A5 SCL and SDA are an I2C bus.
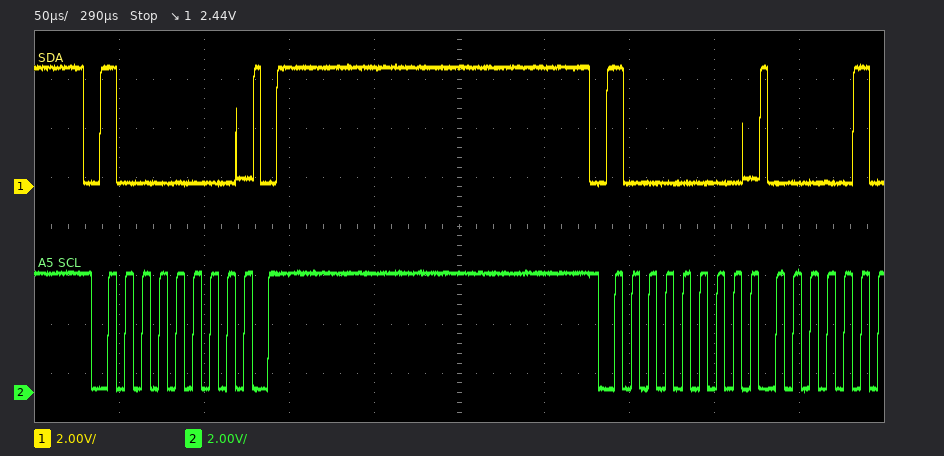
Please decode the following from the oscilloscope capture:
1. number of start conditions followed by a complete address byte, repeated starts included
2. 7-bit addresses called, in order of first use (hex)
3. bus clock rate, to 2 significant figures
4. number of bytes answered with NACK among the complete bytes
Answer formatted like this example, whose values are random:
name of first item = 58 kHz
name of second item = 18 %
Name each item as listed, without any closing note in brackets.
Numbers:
number of start conditions followed by a complete address byte, repeated starts included = 2
7-bit addresses called, in order of first use = 0x40
bus clock rate, to 2 significant figures = 100 kHz
number of bytes answered with NACK among the complete bytes = 0
